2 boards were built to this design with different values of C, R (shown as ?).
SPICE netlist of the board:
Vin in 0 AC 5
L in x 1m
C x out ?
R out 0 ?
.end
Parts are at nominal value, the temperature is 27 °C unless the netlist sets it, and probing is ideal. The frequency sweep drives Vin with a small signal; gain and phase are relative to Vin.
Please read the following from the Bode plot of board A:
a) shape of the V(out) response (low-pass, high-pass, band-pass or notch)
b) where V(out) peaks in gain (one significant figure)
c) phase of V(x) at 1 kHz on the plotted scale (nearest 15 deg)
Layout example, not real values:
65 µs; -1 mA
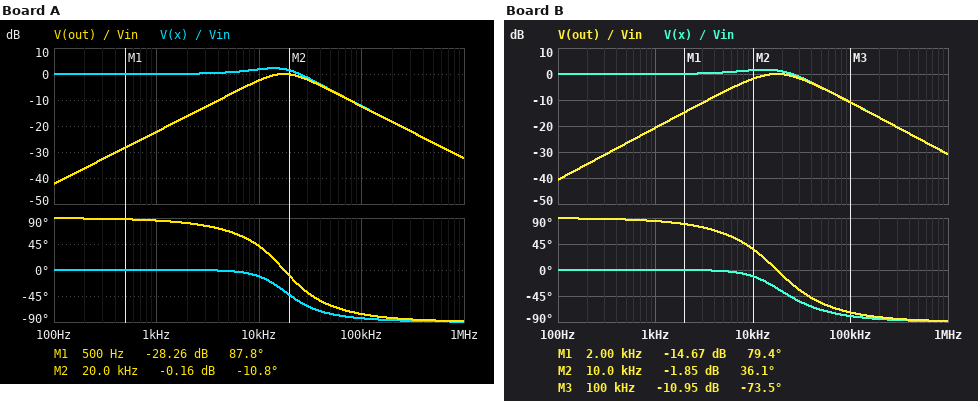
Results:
band-pass; 20 kHz; 0 deg
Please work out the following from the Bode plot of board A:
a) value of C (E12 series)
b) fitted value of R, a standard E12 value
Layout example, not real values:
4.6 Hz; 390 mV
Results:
82 nF; 150 Ω
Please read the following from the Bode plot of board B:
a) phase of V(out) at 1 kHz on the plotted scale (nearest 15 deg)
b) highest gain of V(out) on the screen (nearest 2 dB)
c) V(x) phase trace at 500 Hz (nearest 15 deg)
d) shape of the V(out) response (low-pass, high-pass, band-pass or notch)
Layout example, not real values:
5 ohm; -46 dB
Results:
90 deg; 0 dB; 0 deg; band-pass
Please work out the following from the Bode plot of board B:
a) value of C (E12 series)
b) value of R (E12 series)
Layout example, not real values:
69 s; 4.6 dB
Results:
82 nF; 180 Ω
